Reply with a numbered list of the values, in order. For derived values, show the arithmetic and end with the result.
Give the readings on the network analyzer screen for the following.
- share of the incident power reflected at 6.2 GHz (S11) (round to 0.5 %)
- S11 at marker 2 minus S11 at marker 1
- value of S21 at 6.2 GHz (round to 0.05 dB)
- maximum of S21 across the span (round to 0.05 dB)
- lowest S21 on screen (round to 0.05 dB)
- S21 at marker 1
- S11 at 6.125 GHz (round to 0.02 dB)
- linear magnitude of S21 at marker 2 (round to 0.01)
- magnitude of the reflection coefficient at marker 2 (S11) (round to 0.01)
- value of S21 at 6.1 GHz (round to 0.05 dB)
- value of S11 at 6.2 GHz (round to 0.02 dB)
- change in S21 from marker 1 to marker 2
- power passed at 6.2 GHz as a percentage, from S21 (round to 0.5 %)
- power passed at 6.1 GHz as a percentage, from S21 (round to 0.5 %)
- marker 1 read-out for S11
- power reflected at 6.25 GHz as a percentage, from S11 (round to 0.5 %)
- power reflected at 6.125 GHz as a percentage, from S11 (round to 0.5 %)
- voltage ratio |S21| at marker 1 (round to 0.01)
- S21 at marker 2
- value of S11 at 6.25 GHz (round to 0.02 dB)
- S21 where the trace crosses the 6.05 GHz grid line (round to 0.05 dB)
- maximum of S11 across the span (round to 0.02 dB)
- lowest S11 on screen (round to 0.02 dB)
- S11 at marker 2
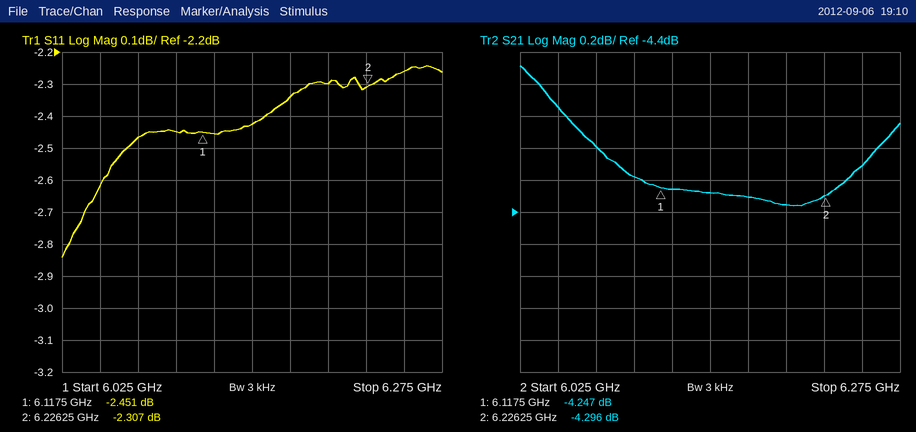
1. 10^(-2.3/10) ≈ 58.9 %, so 59.0 % to the nearest 0.5 %
2. -2.307 − (-2.451) = 0.144 dB
3. -4.35 dB
4. -3.50 dB
5. -4.35 dB
6. -4.247 dB
7. -2.46 dB
8. 10^(-4.296/20) ≈ 0.61
9. 10^(-2.307/20) ≈ 0.77
10. -4.20 dB
11. -2.30 dB
12. -4.296 − (-4.247) = -0.049 dB
13. 10^(-4.35/10) ≈ 36.7 %, so 36.5 % to the nearest 0.5 %
14. 10^(-4.2/10) ≈ 38.0 %
15. -2.451 dB
16. 10^(-2.26/10) ≈ 59.4 %, so 59.5 % to the nearest 0.5 %
17. 10^(-2.46/10) ≈ 56.8 %, so 57.0 % to the nearest 0.5 %
18. 10^(-4.247/20) ≈ 0.61
19. -4.296 dB
20. -2.26 dB
21. -3.75 dB
22. -2.24 dB
23. -2.84 dB
24. -2.307 dB
